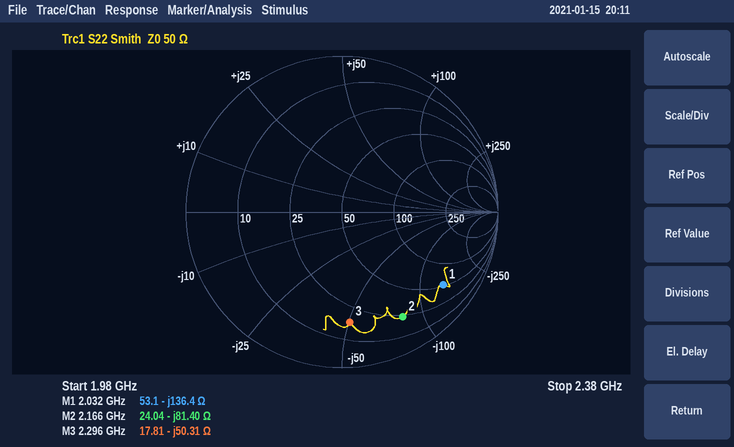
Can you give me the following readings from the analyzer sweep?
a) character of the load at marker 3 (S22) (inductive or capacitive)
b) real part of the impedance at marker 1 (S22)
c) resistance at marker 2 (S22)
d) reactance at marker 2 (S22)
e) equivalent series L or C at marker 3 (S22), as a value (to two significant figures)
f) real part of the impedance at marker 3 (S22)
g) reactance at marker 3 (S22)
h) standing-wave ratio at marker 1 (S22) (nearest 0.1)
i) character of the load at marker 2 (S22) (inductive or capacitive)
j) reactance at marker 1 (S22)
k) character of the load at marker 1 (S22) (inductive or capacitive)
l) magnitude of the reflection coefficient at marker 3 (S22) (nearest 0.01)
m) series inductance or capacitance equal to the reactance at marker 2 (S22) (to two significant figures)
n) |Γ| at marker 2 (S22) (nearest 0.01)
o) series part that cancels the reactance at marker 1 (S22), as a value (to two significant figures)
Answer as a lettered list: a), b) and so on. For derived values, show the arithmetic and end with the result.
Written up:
a) capacitive
b) 53.1 Ω
c) 24.04 Ω
d) -81.40 Ω
e) C = 1/(2π × 2.296 GHz × 50.31 Ω) ≈ 1.4 pF
f) 17.81 Ω
g) -50.31 Ω
h) 8.9
i) capacitive
j) -136.4 Ω
k) capacitive
l) 0.71
m) C = 1/(2π × 2.166 GHz × 81.4 Ω) ≈ 903 fF, so 900 fF to two significant figures
n) 0.78
o) L = 136.4 Ω/(2π × 2.032 GHz) ≈ 11 nH
